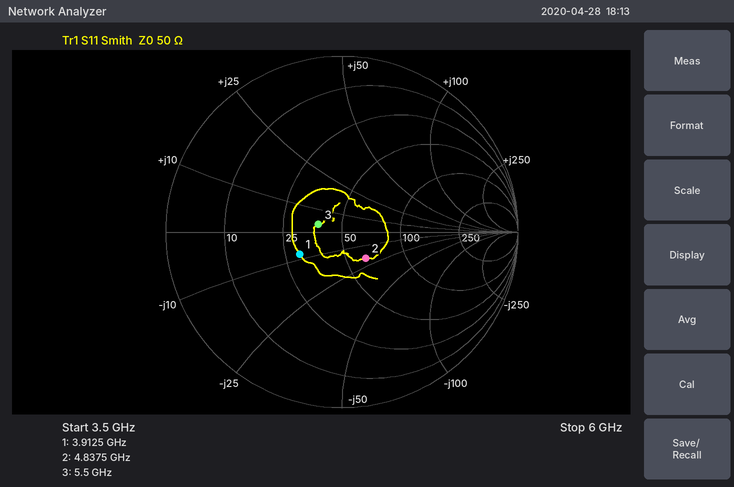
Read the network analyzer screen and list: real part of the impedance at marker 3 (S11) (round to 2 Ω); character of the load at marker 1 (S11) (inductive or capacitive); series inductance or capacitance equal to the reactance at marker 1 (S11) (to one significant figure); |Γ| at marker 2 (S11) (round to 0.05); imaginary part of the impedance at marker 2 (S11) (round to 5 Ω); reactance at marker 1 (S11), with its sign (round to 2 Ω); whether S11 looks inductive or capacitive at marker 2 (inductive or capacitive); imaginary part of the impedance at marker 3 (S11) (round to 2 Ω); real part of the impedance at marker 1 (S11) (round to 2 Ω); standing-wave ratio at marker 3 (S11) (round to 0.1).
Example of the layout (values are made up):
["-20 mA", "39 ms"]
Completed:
["38 Ω", "capacitive", "5 pF", "0.20", "-20 Ω", "-8 Ω", "capacitive", "+4 Ω", "30 Ω", "1.3"]
